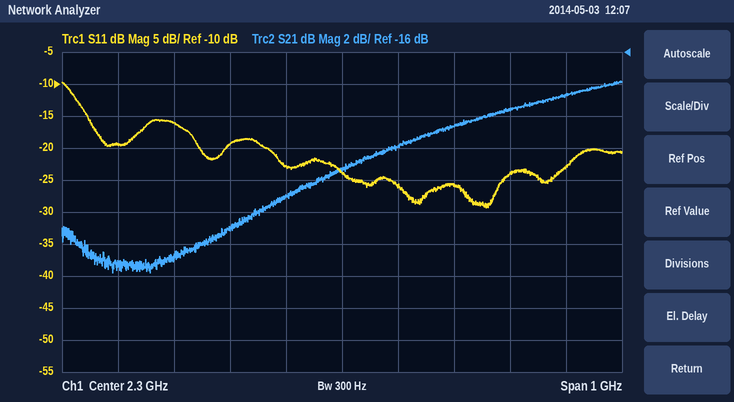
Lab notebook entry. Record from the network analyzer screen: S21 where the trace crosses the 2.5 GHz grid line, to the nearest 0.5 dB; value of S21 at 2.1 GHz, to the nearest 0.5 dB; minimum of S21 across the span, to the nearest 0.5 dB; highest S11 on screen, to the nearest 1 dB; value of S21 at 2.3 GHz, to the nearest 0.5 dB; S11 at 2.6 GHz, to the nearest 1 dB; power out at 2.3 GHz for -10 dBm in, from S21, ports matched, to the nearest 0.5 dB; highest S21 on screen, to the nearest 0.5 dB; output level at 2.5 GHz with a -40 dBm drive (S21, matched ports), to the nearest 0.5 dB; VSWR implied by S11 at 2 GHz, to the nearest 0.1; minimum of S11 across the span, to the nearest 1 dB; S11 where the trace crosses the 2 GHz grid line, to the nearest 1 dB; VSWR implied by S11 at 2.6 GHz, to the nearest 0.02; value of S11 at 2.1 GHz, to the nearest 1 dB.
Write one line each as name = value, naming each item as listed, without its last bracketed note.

S21 where the trace crosses the 2.5 GHz grid line, to the nearest 0.5 dB = -20.5 dB
value of S21 at 2.1 GHz, to the nearest 0.5 dB = -27.0 dB
minimum of S21 across the span, to the nearest 0.5 dB = -30.0 dB
highest S11 on screen, to the nearest 1 dB = -10 dB
value of S21 at 2.3 GHz, to the nearest 0.5 dB = -23.5 dB
S11 at 2.6 GHz, to the nearest 1 dB = -24 dB
power out at 2.3 GHz for -10 dBm in, from S21, ports matched, to the nearest 0.5 dB = -33.5 dBm
highest S21 on screen, to the nearest 0.5 dB = -18.0 dB
output level at 2.5 GHz with a -40 dBm drive (S21, matched ports), to the nearest 0.5 dB = -60.5 dBm
VSWR implied by S11 at 2 GHz, to the nearest 0.1 = 1.4
minimum of S11 across the span, to the nearest 1 dB = -29 dB
S11 where the trace crosses the 2 GHz grid line, to the nearest 1 dB = -16 dB
VSWR implied by S11 at 2.6 GHz, to the nearest 0.02 = 1.14
value of S11 at 2.1 GHz, to the nearest 1 dB = -19 dB
